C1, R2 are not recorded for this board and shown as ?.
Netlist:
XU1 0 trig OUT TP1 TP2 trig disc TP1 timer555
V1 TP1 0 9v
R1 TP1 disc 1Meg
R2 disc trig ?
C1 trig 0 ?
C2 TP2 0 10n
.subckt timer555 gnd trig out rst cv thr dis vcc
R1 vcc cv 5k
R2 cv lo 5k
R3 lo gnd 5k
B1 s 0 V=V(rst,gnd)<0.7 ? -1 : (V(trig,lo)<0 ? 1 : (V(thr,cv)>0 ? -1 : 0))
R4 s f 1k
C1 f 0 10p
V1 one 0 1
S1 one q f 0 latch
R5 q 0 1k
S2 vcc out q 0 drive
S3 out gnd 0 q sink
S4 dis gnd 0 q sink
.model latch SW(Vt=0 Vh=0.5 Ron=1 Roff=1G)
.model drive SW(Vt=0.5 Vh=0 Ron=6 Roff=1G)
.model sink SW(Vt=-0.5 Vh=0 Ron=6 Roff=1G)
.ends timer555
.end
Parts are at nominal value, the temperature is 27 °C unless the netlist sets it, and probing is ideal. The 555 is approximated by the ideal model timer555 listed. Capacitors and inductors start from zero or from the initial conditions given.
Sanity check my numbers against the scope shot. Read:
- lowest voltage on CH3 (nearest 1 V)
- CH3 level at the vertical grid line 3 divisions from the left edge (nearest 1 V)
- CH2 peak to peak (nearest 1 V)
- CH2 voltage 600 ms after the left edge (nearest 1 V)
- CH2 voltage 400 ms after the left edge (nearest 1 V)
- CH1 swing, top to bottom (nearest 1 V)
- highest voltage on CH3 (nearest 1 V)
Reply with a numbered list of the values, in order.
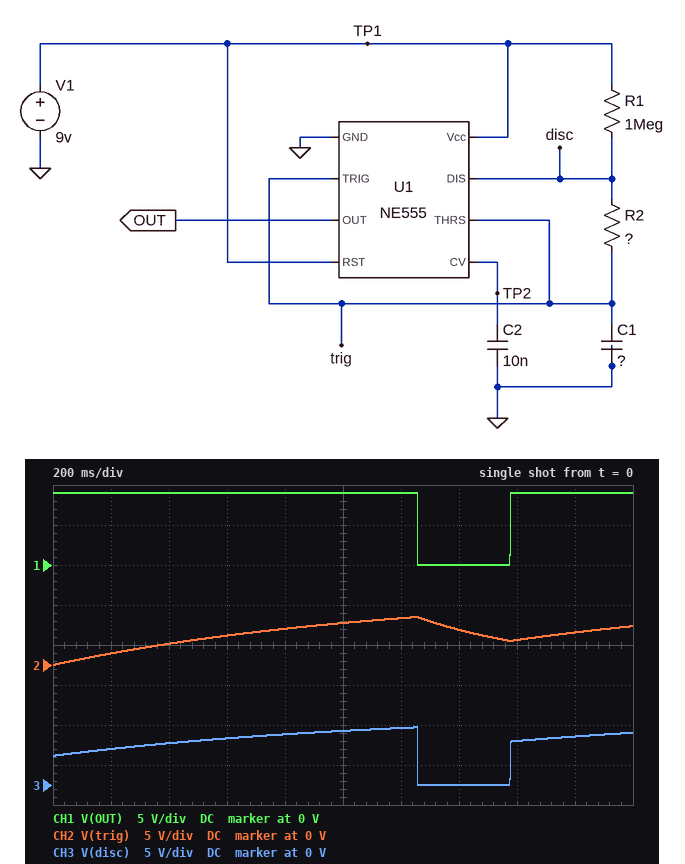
1. 0 V
2. 6 V
3. 6 V
4. 4 V
5. 3 V
6. 9 V
7. 7 V
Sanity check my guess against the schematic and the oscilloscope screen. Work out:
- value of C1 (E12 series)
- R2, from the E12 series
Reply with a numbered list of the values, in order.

1. 680 nF
2. 680 kΩ
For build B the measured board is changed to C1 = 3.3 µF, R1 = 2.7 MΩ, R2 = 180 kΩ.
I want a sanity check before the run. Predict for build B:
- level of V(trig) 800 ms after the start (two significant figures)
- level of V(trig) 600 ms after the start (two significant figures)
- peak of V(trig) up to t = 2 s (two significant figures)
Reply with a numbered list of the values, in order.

1. 730 mV
2. 550 mV
3. 1.7 V
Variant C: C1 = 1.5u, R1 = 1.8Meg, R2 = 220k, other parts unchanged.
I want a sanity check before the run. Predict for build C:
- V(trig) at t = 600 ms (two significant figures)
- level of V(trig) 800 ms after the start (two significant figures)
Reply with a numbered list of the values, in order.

1. 1.6 V
2. 2.1 V
